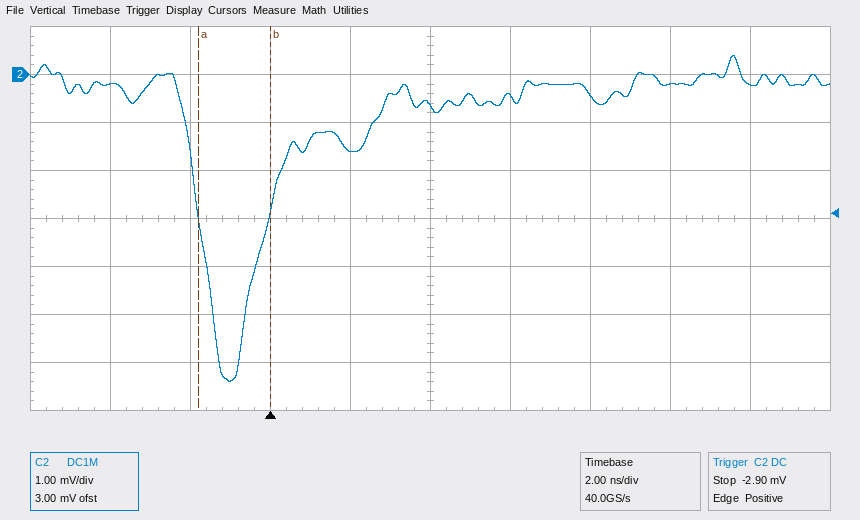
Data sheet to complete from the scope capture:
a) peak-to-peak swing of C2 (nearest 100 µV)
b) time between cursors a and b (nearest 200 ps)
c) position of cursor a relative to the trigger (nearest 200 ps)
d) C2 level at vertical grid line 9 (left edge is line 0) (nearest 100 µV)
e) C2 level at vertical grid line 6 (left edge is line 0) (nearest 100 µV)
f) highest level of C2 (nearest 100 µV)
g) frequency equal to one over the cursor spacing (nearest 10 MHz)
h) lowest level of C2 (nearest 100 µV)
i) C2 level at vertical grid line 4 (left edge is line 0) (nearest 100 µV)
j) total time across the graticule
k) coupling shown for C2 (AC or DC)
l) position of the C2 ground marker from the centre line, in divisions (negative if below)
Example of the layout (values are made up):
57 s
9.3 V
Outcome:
6.8 mV
1.8 ns
-1.8 ns
-200 µV
-500 µV
400 µV
560 MHz
-6.4 mV
-1.6 mV
20 ns
DC
+3.0 div
